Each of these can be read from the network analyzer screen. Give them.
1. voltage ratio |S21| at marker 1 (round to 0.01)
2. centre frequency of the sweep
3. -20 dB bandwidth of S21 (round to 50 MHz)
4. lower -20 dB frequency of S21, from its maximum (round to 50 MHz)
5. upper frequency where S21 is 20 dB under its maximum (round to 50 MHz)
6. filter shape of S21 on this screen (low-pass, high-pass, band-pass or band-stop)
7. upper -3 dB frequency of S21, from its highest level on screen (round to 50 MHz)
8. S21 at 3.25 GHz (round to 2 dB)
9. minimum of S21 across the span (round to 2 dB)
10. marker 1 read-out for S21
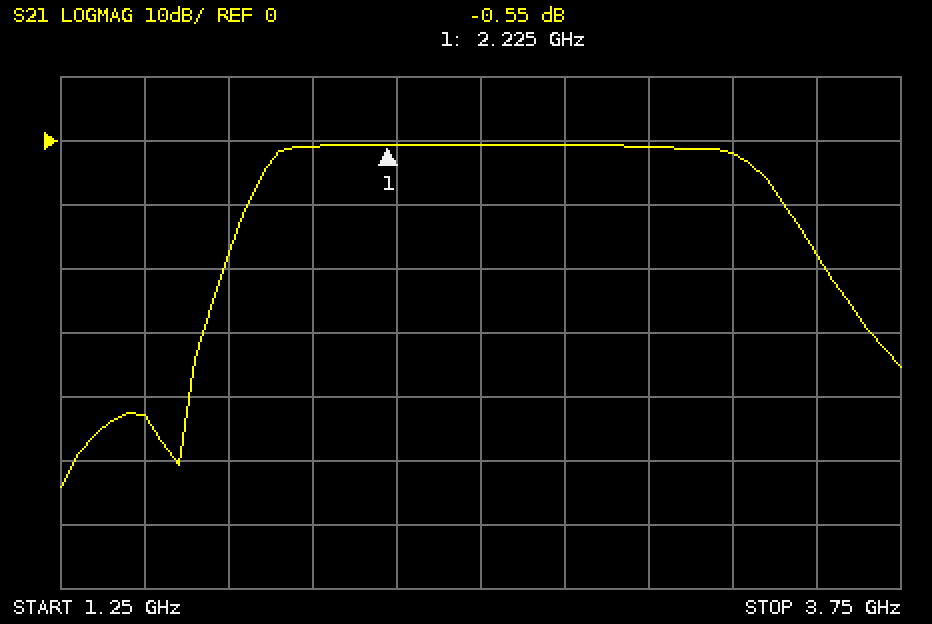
0.94
2.5 GHz
1.80 GHz
1.75 GHz
3.55 GHz
band-pass
3.30 GHz
-2 dB
-54 dB
-0.55 dB
